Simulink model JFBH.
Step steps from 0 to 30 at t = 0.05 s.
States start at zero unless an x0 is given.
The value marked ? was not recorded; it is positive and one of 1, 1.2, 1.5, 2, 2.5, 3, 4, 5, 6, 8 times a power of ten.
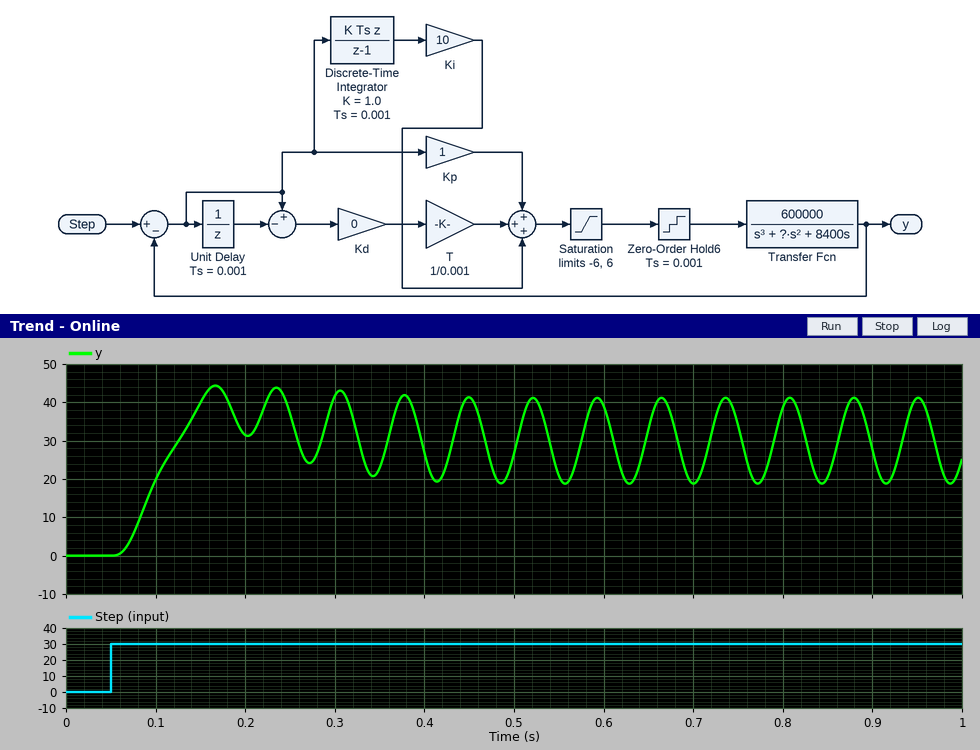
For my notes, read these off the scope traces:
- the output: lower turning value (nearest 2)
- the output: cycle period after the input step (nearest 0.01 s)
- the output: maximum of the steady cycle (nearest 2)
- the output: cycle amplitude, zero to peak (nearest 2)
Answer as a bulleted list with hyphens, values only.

- 18
- 0.07 s
- 42
- 12
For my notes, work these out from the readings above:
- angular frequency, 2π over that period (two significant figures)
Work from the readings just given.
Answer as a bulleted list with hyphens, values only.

- 90 rad/s
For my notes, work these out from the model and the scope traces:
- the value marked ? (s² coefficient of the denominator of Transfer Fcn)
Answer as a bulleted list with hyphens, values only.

- 50
